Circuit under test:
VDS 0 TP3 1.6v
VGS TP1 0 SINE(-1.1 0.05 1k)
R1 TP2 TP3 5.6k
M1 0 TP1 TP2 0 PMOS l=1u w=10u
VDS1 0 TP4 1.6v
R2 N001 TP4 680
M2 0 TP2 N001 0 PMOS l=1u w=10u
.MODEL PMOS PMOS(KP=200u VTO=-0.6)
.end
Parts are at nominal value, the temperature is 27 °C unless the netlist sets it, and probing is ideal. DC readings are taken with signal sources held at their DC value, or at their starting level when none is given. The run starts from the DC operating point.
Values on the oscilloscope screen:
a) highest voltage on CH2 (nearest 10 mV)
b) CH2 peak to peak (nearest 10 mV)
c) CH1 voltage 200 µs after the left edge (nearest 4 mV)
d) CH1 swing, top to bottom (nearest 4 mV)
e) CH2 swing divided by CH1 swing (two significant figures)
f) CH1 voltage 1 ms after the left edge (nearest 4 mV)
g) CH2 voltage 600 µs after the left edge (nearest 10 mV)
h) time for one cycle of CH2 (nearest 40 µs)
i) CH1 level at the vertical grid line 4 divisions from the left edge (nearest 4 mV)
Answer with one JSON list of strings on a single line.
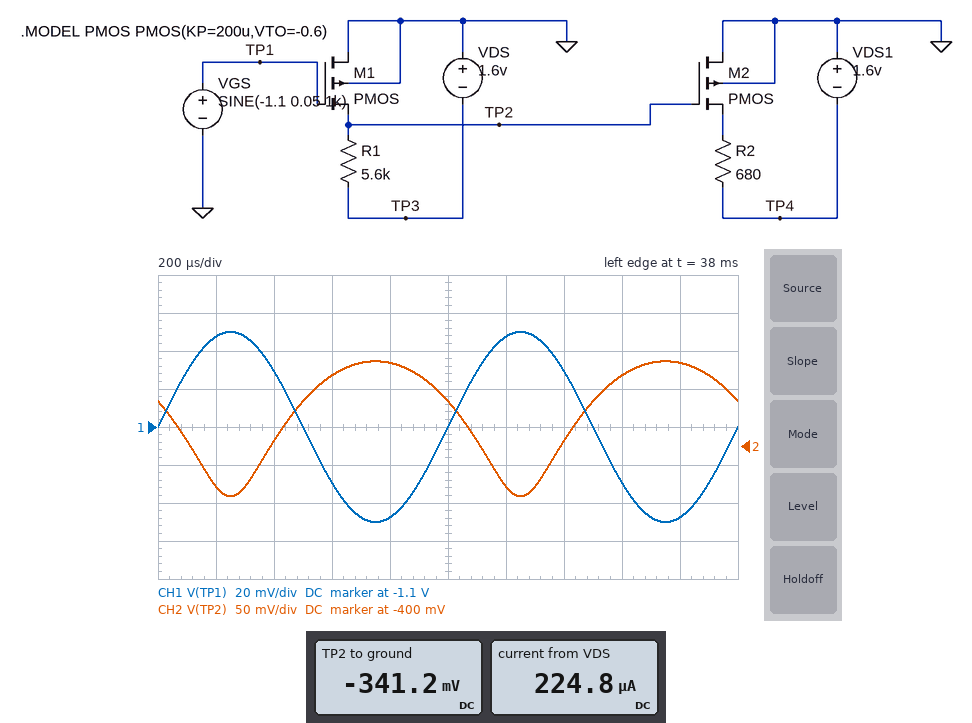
["-290 mV", "180 mV", "-1.052 V", "100 mV", "1.8", "-1.100 V", "-310 mV", "1.00 ms", "-1.148 V"]
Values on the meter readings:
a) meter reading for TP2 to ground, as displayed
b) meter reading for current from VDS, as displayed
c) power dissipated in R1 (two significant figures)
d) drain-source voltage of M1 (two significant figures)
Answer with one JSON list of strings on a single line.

["-341.2 mV", "224.8 µA", "280 µW", "340 mV"]
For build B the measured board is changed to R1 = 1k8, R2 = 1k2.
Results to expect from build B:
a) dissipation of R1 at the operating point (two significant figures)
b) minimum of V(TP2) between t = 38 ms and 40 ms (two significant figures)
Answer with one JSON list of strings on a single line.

["110 µW", "-1.2 V"]
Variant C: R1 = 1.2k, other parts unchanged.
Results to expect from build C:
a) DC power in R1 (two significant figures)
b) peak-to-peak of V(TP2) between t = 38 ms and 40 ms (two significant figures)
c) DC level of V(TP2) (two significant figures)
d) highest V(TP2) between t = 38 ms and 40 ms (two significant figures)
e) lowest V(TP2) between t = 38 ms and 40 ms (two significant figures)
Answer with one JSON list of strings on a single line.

["75 µW", "120 mV", "-1.3 V", "-1.2 V", "-1.4 V"]
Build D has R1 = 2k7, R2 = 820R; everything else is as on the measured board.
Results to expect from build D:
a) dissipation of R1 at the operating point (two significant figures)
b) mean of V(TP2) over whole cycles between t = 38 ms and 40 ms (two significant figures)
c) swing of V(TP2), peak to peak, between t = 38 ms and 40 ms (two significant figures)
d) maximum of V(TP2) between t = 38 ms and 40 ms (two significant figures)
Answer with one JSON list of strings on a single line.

["170 µW", "-920 mV", "270 mV", "-780 mV"]
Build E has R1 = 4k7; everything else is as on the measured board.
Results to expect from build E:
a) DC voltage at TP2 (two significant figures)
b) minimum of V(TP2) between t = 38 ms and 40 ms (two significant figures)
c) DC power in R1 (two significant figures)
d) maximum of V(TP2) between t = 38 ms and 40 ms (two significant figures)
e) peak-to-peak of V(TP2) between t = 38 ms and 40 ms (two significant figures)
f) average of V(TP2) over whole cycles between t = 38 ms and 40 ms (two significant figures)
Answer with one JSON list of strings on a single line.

["-440 mV", "-650 mV", "290 µW", "-360 mV", "290 mV", "-480 mV"]
